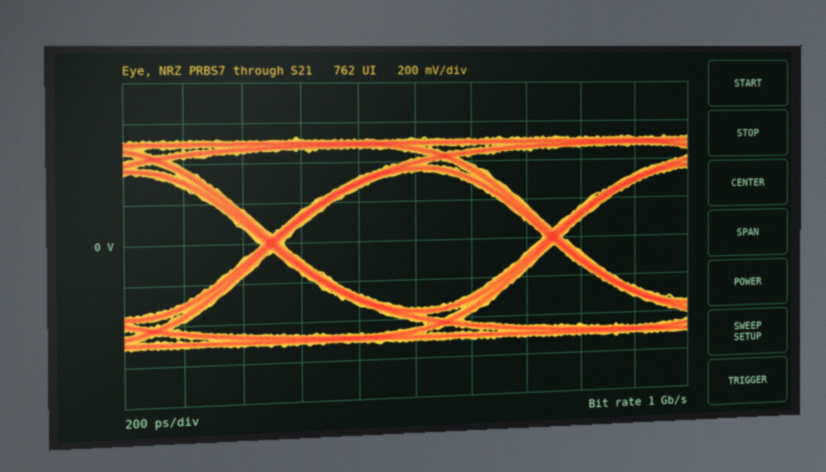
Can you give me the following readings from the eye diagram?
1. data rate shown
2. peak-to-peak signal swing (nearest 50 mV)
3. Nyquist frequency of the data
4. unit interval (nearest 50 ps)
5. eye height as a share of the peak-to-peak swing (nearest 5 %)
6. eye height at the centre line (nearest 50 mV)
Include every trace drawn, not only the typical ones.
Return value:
1 Gb/s
1.05 V
500 MHz
1.00 ns
65 %
700 mV
